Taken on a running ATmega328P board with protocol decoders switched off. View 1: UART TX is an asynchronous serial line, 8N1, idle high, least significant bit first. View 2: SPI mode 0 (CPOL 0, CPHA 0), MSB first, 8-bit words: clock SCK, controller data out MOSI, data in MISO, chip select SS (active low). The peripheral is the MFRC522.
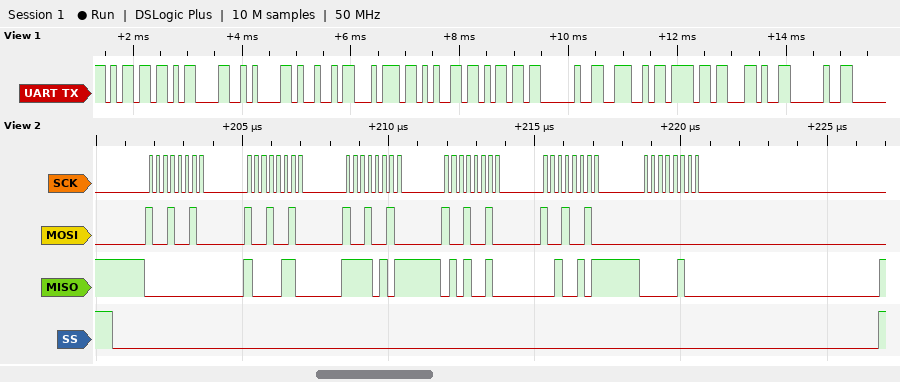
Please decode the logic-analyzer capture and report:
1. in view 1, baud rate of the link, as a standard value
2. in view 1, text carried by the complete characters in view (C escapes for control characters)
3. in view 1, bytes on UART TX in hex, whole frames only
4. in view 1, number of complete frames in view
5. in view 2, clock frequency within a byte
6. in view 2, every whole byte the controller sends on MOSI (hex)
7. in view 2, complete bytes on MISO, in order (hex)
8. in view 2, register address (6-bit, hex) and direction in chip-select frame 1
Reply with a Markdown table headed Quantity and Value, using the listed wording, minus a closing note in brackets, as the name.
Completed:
| Quantity | Value |
|---|---|
| in view 1, baud rate of the link, as a standard value | 9600 baud |
| in view 1, text carried by the complete characters in view | "m\r\nItem No, " |
| in view 1, bytes on UART TX in hex, whole frames only | 6D 0D 0A 49 74 65 6D 20 4E 6F 2C 20 |
| in view 1, number of complete frames in view | 12 |
| in view 2, clock frequency within a byte | 4 MHz |
| in view 2, every whole byte the controller sends on MOSI | 92 92 92 92 92 00 |
| in view 2, complete bytes on MISO, in order | 00 86 F5 52 25 04 |
| in view 2, register address (6-bit, hex) and direction in chip-select frame 1 | 0x09 read |
